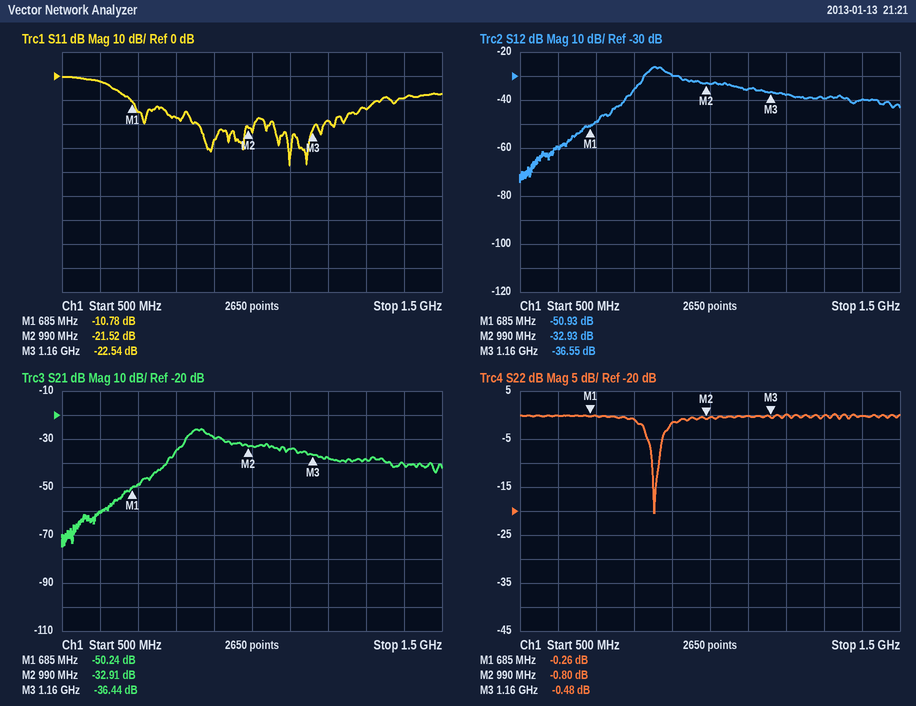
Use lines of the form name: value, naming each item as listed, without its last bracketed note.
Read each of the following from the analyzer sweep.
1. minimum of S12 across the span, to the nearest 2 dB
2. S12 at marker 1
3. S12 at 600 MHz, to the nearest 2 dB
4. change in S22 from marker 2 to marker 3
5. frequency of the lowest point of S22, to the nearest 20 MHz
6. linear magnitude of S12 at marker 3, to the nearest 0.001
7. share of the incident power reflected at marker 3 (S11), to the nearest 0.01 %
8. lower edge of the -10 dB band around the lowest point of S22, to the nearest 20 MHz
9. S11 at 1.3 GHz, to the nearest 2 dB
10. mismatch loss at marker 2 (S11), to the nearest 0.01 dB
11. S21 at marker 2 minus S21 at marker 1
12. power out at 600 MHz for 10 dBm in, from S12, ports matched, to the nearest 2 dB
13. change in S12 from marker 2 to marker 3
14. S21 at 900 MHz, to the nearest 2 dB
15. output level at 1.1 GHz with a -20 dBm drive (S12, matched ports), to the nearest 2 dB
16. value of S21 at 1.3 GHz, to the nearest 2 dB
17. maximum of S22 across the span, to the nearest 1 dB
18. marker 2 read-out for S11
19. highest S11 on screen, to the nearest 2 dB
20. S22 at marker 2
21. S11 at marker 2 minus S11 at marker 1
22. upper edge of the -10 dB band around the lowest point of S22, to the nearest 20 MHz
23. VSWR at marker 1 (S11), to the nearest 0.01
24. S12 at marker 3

minimum of S12 across the span, to the nearest 2 dB: -74 dB
S12 at marker 1: -50.93 dB
S12 at 600 MHz, to the nearest 2 dB: -60 dB
change in S22 from marker 2 to marker 3: 0.32 dB
frequency of the lowest point of S22, to the nearest 20 MHz: 860 MHz
linear magnitude of S12 at marker 3, to the nearest 0.001: 0.015
share of the incident power reflected at marker 3 (S11), to the nearest 0.01 %: 0.56 %
lower edge of the -10 dB band around the lowest point of S22, to the nearest 20 MHz: 840 MHz
S11 at 1.3 GHz, to the nearest 2 dB: -14 dB
mismatch loss at marker 2 (S11), to the nearest 0.01 dB: 0.03 dB
S21 at marker 2 minus S21 at marker 1: 17.33 dB
power out at 600 MHz for 10 dBm in, from S12, ports matched, to the nearest 2 dB: -50 dBm
change in S12 from marker 2 to marker 3: -3.62 dB
S21 at 900 MHz, to the nearest 2 dB: -30 dB
output level at 1.1 GHz with a -20 dBm drive (S12, matched ports), to the nearest 2 dB: -56 dBm
value of S21 at 1.3 GHz, to the nearest 2 dB: -38 dB
maximum of S22 across the span, to the nearest 1 dB: 0 dB
marker 2 read-out for S11: -21.52 dB
highest S11 on screen, to the nearest 2 dB: 0 dB
S22 at marker 2: -0.80 dB
S11 at marker 2 minus S11 at marker 1: -10.74 dB
upper edge of the -10 dB band around the lowest point of S22, to the nearest 20 MHz: 860 MHz
VSWR at marker 1 (S11), to the nearest 0.01: 1.81
S12 at marker 3: -36.55 dB
